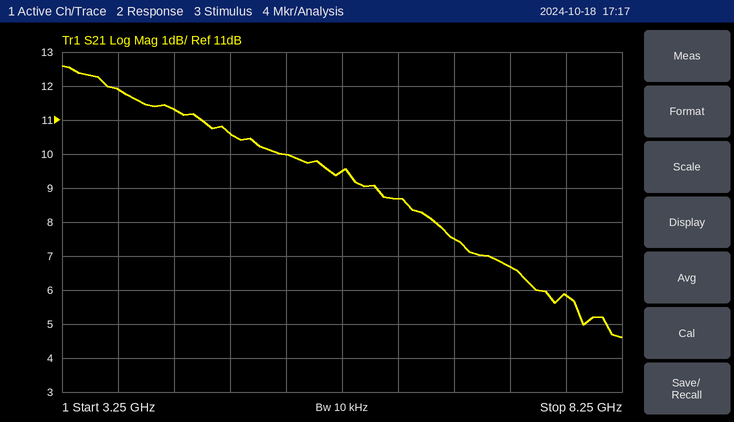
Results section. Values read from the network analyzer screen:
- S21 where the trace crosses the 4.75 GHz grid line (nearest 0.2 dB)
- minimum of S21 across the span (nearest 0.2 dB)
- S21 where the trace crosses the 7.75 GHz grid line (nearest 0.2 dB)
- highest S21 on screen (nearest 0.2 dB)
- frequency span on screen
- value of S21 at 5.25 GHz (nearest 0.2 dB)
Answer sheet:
10.6 dB
4.6 dB
5.8 dB
12.6 dB
5 GHz
10.0 dB
